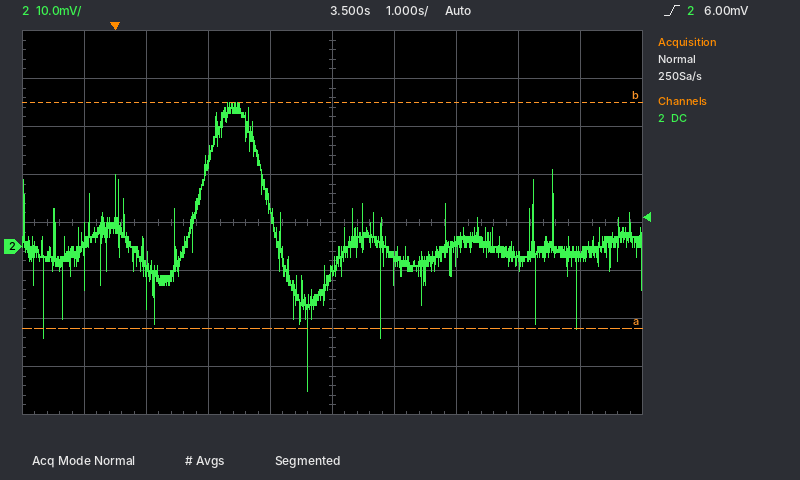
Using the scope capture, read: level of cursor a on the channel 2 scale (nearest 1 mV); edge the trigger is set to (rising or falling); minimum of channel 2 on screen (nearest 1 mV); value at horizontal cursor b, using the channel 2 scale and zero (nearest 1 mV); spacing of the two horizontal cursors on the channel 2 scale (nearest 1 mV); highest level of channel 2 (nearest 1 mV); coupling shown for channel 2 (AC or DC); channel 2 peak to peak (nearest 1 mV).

-17 mV
rising
-30 mV
30 mV
47 mV
30 mV
DC
60 mV
